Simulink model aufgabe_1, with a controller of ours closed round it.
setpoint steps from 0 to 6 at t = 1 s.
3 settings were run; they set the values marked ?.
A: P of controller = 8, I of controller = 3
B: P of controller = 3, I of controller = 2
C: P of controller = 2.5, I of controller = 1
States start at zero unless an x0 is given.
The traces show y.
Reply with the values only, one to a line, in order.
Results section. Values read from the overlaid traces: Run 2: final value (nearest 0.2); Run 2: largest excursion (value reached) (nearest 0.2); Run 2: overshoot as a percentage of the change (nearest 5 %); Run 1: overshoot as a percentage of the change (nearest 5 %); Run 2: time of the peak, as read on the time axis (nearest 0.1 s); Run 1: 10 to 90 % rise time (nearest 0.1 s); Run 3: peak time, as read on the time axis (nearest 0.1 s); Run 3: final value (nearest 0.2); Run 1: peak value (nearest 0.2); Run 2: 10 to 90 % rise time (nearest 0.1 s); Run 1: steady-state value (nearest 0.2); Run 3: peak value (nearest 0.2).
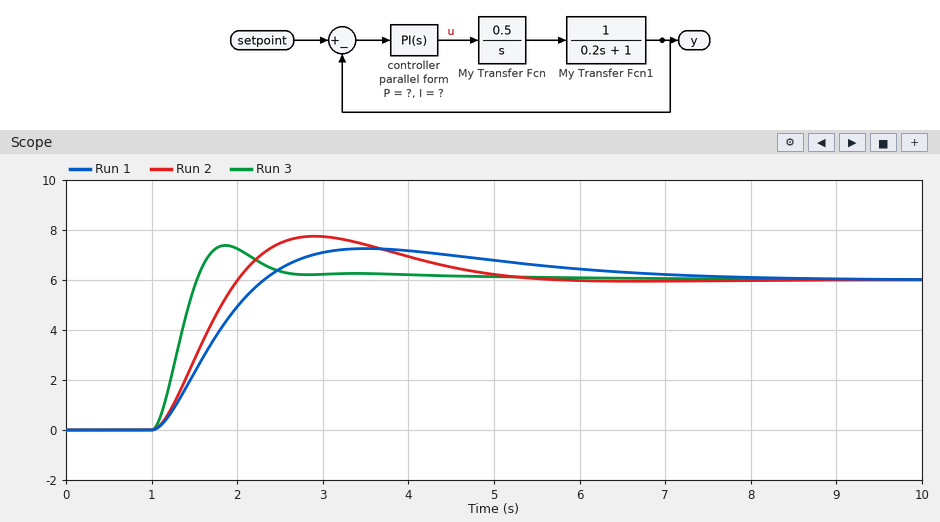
6.0
7.8
30 %
20 %
2.9 s
0.9 s
1.9 s
6.0
7.2
0.7 s
6.0
7.4
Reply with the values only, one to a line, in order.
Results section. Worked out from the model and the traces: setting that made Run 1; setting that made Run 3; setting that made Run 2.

C
A
B
